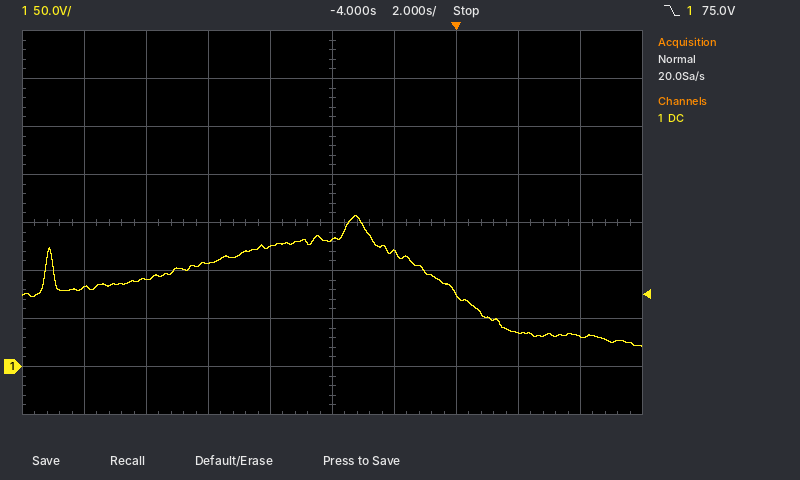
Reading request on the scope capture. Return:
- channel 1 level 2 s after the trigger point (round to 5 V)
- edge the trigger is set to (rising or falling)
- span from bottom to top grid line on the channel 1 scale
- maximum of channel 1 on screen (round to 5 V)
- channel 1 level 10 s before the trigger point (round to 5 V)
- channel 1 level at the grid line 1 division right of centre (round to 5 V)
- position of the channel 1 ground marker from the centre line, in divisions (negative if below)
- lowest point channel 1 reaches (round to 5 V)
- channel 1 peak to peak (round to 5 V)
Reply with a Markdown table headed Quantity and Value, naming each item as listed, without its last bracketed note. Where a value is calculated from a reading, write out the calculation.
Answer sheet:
| Quantity | Value |
|---|---|
| channel 1 level 2 s after the trigger point | 35 V |
| edge the trigger is set to | falling |
| span from bottom to top grid line on the channel 1 scale | 400 V |
| maximum of channel 1 on screen | 155 V |
| channel 1 level 10 s before the trigger point | 90 V |
| channel 1 level at the grid line 1 division right of centre | 120 V |
| position of the channel 1 ground marker from the centre line, in divisions | -3.0 div |
| lowest point channel 1 reaches | 20 V |
| channel 1 peak to peak | 155 V − (20 V) = 135 V |
